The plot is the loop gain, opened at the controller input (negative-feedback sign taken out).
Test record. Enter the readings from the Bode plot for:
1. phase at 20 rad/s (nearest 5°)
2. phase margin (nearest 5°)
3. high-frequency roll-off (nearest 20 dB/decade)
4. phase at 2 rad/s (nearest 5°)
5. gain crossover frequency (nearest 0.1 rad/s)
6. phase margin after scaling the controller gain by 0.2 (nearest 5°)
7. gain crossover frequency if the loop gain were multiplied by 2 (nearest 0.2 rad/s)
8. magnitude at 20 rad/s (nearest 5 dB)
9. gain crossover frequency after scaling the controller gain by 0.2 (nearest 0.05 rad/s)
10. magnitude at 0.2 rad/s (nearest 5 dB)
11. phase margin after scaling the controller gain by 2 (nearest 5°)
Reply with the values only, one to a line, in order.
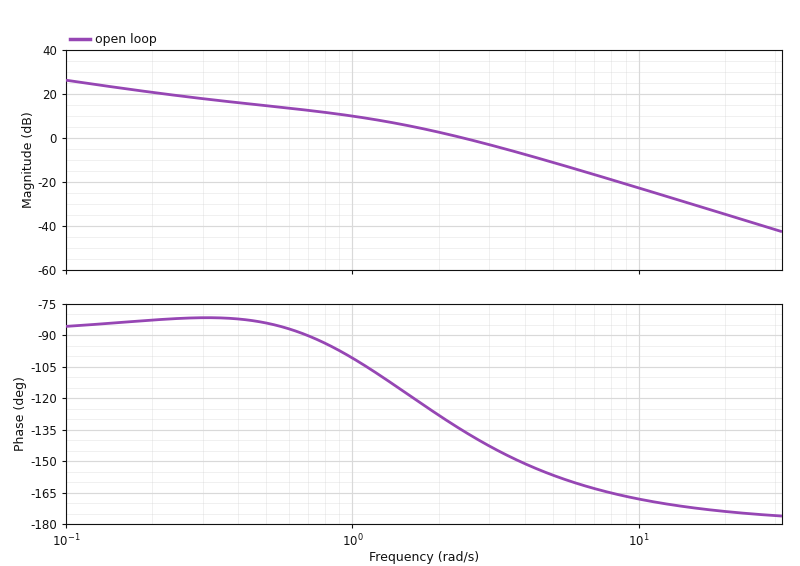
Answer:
-175°
45°
-40 dB/decade
-130°
2.4 rad/s
95°
3.6 rad/s
-35 dB
0.55 rad/s
20 dB
30°
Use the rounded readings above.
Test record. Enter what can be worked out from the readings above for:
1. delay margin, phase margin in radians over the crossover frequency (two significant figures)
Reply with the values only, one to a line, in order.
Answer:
0.33 s
